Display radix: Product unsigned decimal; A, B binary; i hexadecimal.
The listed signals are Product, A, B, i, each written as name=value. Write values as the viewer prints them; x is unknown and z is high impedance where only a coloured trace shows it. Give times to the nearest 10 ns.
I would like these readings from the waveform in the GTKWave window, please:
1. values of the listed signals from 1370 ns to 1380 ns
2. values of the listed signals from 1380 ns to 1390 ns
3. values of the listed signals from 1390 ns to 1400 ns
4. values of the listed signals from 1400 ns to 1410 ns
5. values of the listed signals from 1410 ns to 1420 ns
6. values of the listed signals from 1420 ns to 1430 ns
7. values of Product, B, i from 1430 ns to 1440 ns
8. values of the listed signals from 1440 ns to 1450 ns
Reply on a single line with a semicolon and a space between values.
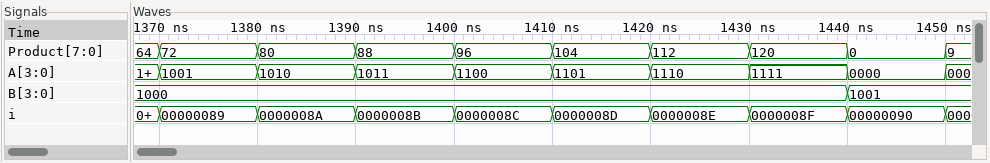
Product=72, A=1001, B=1000, i=00000089; Product=80, A=1010, B=1000, i=0000008A; Product=88, A=1011, B=1000, i=0000008B; Product=96, A=1100, B=1000, i=0000008C; Product=104, A=1101, B=1000, i=0000008D; Product=112, A=1110, B=1000, i=0000008E; Product=120, B=1000, i=0000008F; Product=0, A=0000, B=1001, i=00000090
